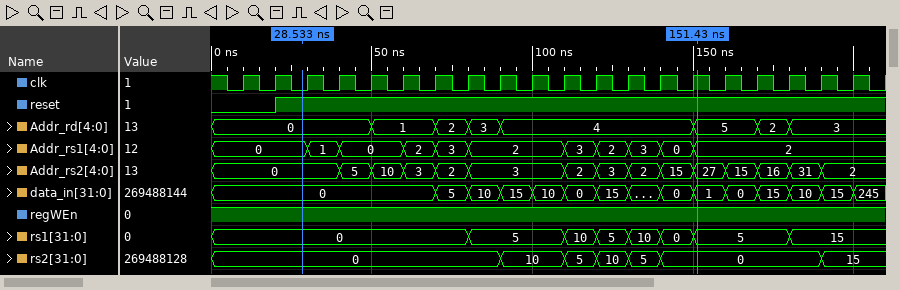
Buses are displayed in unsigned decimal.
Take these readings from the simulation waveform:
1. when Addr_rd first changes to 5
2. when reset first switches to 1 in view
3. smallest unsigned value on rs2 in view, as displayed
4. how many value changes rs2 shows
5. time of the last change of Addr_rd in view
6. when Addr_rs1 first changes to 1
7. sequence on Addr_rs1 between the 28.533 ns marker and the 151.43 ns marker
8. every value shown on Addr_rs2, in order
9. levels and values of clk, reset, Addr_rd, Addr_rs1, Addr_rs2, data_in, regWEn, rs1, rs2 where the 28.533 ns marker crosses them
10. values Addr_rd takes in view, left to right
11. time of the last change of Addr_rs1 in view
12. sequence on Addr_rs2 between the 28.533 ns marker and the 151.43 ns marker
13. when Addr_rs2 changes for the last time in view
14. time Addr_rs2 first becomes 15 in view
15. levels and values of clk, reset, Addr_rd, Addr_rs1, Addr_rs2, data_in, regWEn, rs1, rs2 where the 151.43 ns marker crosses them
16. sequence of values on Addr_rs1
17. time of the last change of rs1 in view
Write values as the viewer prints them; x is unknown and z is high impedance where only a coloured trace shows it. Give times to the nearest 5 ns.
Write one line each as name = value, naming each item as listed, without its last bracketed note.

when Addr_rd first changes to 5 = 150 ns
when reset first switches to 1 in view = 20 ns
smallest unsigned value on rs2 in view, as displayed = 0
how many value changes rs2 shows = 6
time of the last change of Addr_rd in view = 180 ns
when Addr_rs1 first changes to 1 = 30 ns
sequence on Addr_rs1 between the 28.533 ns marker and the 151.43 ns marker = 0, 1, 0, 2, 3, 2, 3, 2, 3, 0, 2
every value shown on Addr_rs2, in order = 0, 5, 10, 3, 2, 3, 2, 3, 2, 15, 27, 15, 16, 31, 2
levels and values of clk, reset, Addr_rd, Addr_rs1, Addr_rs2, data_in, regWEn, rs1, rs2 where the 28.533 ns marker crosses them = clk=0, reset=1, Addr_rd=0, Addr_rs1=0, Addr_rs2=0, data_in=0, regWEn=1, rs1=0, rs2=0
values Addr_rd takes in view, left to right = 0, 1, 2, 3, 4, 5, 2, 3
time of the last change of Addr_rs1 in view = 150 ns
sequence on Addr_rs2 between the 28.533 ns marker and the 151.43 ns marker = 0, 5, 10, 3, 2, 3, 2, 3, 2, 15, 27
when Addr_rs2 changes for the last time in view = 190 ns
time Addr_rs2 first becomes 15 in view = 140 ns
levels and values of clk, reset, Addr_rd, Addr_rs1, Addr_rs2, data_in, regWEn, rs1, rs2 where the 151.43 ns marker crosses them = clk=1, reset=1, Addr_rd=5, Addr_rs1=2, Addr_rs2=27, data_in=1, regWEn=1, rs1=5, rs2=0
sequence of values on Addr_rs1 = 0, 1, 0, 2, 3, 2, 3, 2, 3, 0, 2
time of the last change of rs1 in view = 180 ns
